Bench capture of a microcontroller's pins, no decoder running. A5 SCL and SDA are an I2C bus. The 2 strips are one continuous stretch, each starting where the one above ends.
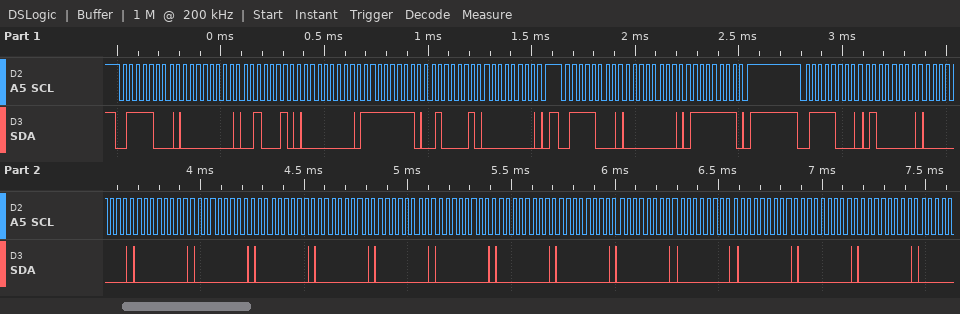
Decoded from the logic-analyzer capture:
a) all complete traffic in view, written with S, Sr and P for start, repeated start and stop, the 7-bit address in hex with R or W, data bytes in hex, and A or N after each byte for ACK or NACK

S 3CW A 00 A 22 A 00 A FF A 21 A 00 A P S 3CW A 00 A 7F A P S 3CW A 40 A 00 A 00 A 00 A 00 A 00 A 00 A 00 A 00 A 00 A 00 A 00 A 00 A 00 A 00 A
